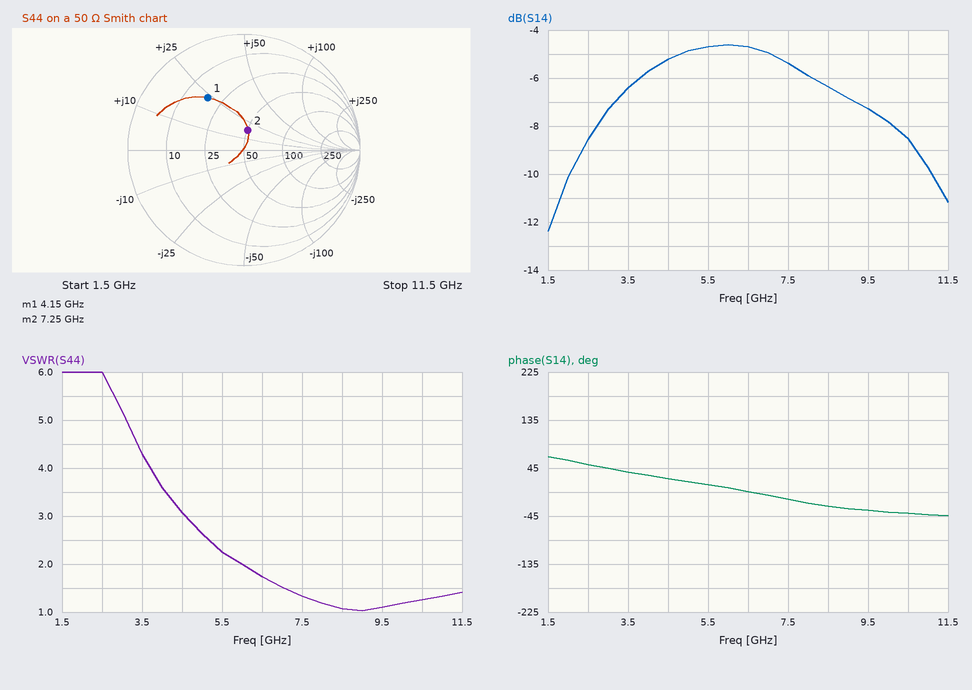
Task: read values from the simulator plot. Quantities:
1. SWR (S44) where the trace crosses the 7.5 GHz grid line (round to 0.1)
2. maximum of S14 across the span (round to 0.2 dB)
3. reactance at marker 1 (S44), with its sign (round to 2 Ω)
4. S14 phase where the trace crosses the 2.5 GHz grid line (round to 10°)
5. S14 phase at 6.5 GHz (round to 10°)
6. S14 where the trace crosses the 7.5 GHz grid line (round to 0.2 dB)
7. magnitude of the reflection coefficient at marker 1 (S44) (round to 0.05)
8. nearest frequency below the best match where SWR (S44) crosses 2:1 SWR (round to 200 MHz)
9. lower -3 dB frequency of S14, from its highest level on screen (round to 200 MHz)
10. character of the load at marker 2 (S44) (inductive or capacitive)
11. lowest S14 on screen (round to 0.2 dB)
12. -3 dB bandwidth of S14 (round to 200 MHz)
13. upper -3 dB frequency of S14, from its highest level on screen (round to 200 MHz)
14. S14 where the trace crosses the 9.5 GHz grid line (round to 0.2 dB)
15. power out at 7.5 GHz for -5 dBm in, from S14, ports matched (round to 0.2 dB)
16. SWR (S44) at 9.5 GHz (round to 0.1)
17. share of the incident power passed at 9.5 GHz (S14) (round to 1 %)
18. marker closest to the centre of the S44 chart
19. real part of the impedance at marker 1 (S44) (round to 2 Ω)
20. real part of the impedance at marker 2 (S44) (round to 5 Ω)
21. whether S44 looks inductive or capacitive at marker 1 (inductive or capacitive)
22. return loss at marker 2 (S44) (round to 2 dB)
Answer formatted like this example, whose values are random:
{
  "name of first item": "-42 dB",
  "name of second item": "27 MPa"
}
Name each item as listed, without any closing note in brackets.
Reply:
{
  "SWR (S44) where the trace crosses the 7.5 GHz grid line": "1.3",
  "maximum of S14 across the span": "-4.6 dB",
  "reactance at marker 1 (S44), with its sign": "+24 Ω",
  "S14 phase where the trace crosses the 2.5 GHz grid line": "50°",
  "S14 phase at 6.5 GHz": "0°",
  "S14 where the trace crosses the 7.5 GHz grid line": "-5.4 dB",
  "magnitude of the reflection coefficient at marker 1 (S44)": "0.55",
  "nearest frequency below the best match where SWR (S44) crosses 2:1 SWR": "6.0 GHz",
  "lower -3 dB frequency of S14, from its highest level on screen": "2.8 GHz",
  "character of the load at marker 2 (S44)": "inductive",
  "lowest S14 on screen": "-12.4 dB",
  "-3 dB bandwidth of S14": "7.0 GHz",
  "upper -3 dB frequency of S14, from its highest level on screen": "9.8 GHz",
  "S14 where the trace crosses the 9.5 GHz grid line": "-7.2 dB",
  "power out at 7.5 GHz for -5 dBm in, from S14, ports matched": "-10.4 dBm",
  "SWR (S44) at 9.5 GHz": "1.1",
  "share of the incident power passed at 9.5 GHz (S14)": "19 %",
  "marker closest to the centre of the S44 chart": "marker 2",
  "real part of the impedance at marker 1 (S44)": "18 Ω",
  "real part of the impedance at marker 2 (S44)": "50 Ω",
  "whether S44 looks inductive or capacitive at marker 1": "inductive",
  "return loss at marker 2 (S44)": "16 dB"
}
